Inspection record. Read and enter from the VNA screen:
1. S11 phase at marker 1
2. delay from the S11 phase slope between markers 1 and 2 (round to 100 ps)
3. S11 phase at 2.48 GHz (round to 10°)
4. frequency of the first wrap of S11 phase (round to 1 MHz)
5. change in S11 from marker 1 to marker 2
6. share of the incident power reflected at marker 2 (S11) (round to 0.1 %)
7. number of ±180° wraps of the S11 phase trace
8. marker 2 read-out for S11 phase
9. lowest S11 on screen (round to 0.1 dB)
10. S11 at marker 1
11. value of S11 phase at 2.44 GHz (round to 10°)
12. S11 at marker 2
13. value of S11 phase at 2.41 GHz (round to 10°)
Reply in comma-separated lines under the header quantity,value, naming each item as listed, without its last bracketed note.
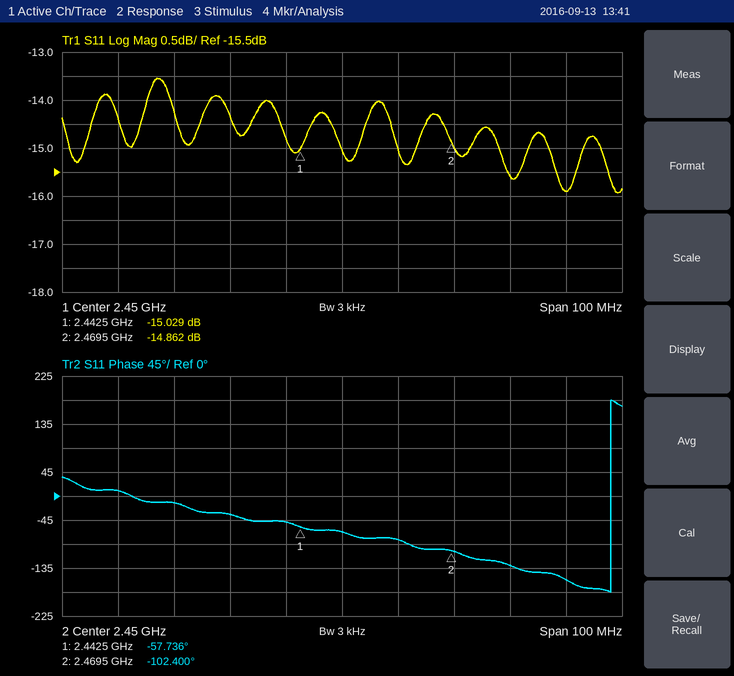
quantity,value
S11 phase at marker 1,-57.736°
delay from the S11 phase slope between markers 1 and 2,4.6 ns
S11 phase at 2.48 GHz,-130°
frequency of the first wrap of S11 phase,2.498 GHz
change in S11 from marker 1 to marker 2,0.167 dB
share of the incident power reflected at marker 2 (S11),3.3 %
number of ±180° wraps of the S11 phase trace,1
marker 2 read-out for S11 phase,-102.400°
lowest S11 on screen,-15.9 dB
S11 at marker 1,-15.029 dB
value of S11 phase at 2.44 GHz,-50°
S11 at marker 2,-14.862 dB
value of S11 phase at 2.41 GHz,10°
